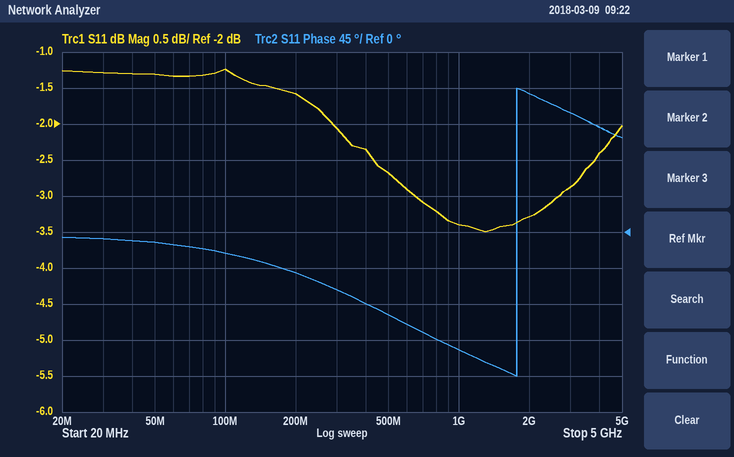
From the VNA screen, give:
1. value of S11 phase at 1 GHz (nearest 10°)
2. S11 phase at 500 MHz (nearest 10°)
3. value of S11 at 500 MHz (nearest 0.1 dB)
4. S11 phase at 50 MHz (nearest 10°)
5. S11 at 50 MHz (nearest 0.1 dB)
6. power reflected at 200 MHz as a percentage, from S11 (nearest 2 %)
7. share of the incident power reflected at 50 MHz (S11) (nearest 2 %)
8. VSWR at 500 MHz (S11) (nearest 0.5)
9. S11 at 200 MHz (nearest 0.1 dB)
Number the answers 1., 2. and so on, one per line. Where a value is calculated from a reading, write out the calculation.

1. -150°
2. -100°
3. -2.7 dB
4. -10°
5. -1.3 dB
6. 10^(-1.6/10) ≈ 69.2 %, so 70 % to the nearest 2 %
7. 10^(-1.3/10) ≈ 74 %
8. |Γ| = 10^(-2.7/20) = 0.7328; VSWR = (1 + 0.7328)/(1 − 0.7328) ≈ 6.5
9. -1.6 dB
